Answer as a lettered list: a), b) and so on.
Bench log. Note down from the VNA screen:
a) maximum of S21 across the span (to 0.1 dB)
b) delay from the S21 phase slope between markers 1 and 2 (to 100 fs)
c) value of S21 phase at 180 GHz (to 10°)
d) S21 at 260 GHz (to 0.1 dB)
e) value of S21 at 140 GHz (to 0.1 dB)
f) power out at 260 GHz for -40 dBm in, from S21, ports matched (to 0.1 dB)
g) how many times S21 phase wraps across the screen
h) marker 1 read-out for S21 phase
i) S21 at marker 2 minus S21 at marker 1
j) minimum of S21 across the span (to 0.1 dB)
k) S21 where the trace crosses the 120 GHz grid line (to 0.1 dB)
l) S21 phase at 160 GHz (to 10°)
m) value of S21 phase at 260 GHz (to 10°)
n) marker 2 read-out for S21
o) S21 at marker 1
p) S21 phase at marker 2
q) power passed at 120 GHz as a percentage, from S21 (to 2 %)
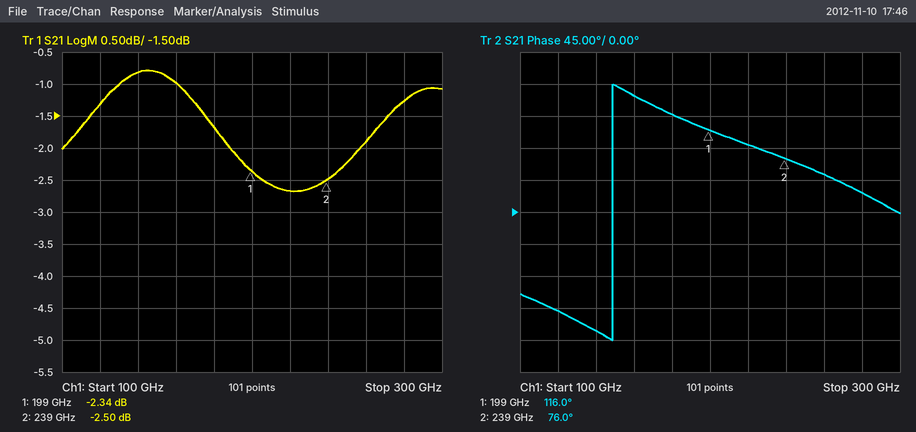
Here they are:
a) -0.8 dB
b) 2.8 ps
c) 140°
d) -1.9 dB
e) -0.8 dB
f) -41.9 dBm
g) 1
h) 116.0°
i) -0.16 dB
j) -2.7 dB
k) -1.3 dB
l) 160°
m) 50°
n) -2.50 dB
o) -2.34 dB
p) 76.0°
q) 74 %
